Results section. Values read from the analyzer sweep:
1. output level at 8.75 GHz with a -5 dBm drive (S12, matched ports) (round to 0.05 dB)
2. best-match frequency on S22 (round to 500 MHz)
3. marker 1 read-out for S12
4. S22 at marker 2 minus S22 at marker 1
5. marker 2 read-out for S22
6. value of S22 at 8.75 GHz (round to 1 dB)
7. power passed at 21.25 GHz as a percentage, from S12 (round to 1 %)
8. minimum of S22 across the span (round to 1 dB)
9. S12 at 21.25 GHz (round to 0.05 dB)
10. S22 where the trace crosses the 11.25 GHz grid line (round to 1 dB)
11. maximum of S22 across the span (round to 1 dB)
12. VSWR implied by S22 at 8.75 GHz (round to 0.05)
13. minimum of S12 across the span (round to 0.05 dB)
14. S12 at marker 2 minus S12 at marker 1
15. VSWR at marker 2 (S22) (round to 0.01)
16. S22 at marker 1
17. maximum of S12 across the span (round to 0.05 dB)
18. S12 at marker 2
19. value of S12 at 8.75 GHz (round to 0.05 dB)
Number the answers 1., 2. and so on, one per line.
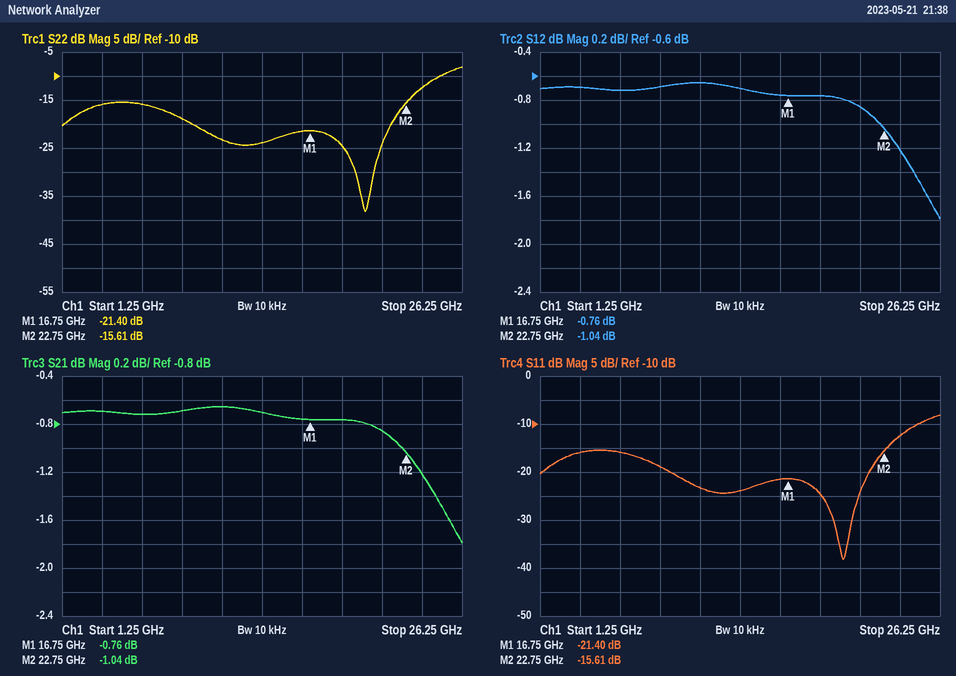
1. -5.70 dBm
2. 20.0 GHz
3. -0.76 dB
4. 5.79 dB
5. -15.61 dB
6. -19 dB
7. 82 %
8. -38 dB
9. -0.85 dB
10. -23 dB
11. -8 dB
12. 1.25
13. -1.80 dB
14. -0.28 dB
15. 1.40
16. -21.40 dB
17. -0.65 dB
18. -1.04 dB
19. -0.70 dB
